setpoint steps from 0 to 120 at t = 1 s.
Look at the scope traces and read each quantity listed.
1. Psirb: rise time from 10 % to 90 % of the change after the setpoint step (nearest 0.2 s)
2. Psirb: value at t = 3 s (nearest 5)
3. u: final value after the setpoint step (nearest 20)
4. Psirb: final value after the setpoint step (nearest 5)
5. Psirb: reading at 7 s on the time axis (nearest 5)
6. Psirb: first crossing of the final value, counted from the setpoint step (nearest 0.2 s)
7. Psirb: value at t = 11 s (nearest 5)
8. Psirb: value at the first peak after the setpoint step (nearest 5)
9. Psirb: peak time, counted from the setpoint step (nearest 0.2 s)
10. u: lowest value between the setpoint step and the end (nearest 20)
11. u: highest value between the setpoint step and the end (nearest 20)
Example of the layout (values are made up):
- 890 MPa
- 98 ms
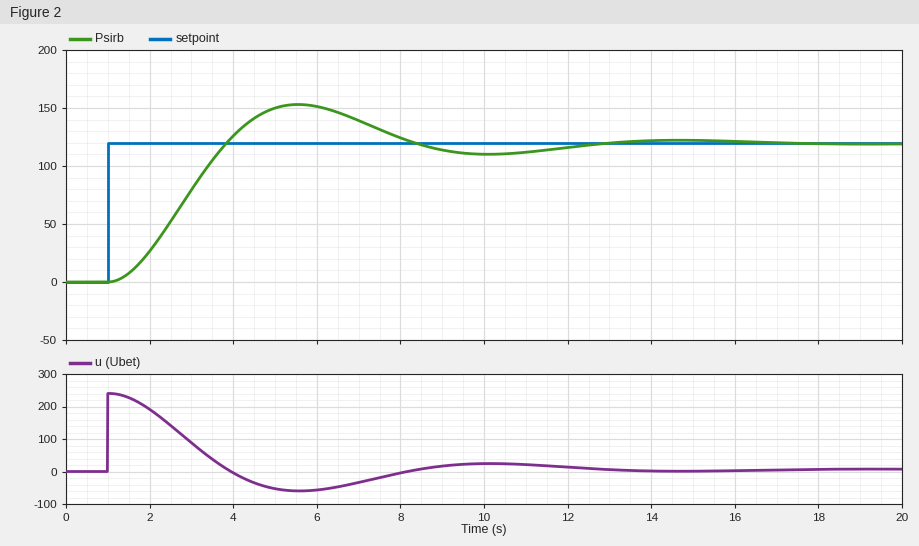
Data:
- 2.0 s
- 80
- 0
- 120
- 140
- 2.8 s
- 110
- 155
- 4.6 s
- -60
- 240
